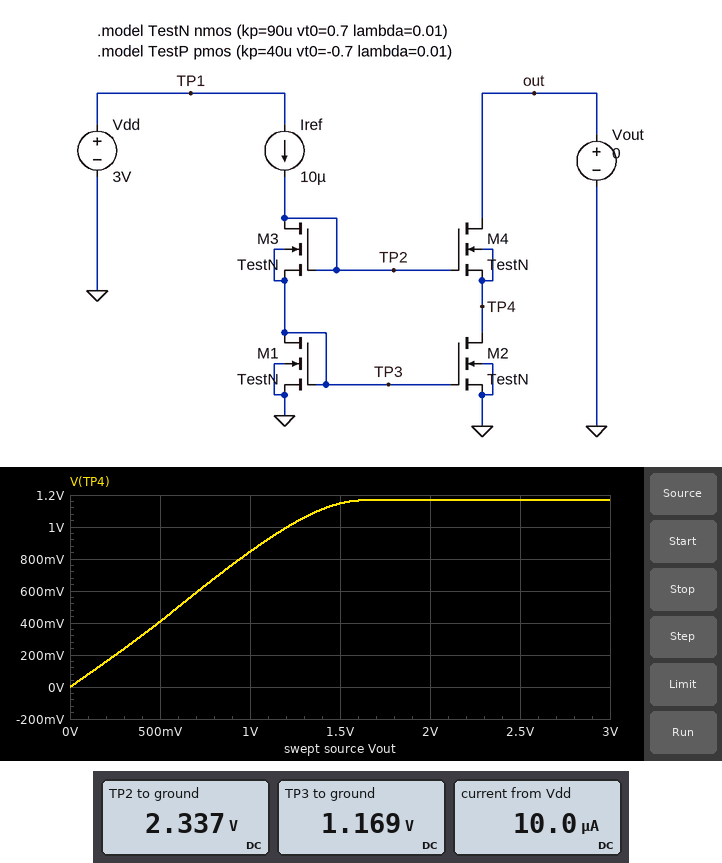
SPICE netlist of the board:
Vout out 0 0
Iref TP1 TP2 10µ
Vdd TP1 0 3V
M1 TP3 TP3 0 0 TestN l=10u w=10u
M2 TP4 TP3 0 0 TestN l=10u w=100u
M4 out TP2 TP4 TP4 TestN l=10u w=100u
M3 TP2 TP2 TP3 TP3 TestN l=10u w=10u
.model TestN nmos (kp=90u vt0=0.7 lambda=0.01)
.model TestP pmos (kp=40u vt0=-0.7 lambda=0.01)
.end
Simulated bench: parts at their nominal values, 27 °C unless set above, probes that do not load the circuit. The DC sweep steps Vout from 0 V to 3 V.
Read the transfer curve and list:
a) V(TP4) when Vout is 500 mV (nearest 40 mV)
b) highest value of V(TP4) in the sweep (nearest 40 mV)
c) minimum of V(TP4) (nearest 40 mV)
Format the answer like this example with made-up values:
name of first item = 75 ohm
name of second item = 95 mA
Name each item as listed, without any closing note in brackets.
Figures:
V(TP4) when Vout is 500 mV = 400 mV
highest value of V(TP4) in the sweep = 1.16 V
minimum of V(TP4) = 0 V
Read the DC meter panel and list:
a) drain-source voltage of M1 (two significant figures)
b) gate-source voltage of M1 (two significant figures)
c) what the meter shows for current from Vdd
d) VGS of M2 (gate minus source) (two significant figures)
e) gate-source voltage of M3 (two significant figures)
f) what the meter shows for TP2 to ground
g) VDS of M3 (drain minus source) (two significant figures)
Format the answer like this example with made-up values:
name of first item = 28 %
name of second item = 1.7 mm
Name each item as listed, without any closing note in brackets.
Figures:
drain-source voltage of M1 = 1.2 V
gate-source voltage of M1 = 1.2 V
what the meter shows for current from Vdd = 10.0 µA
VGS of M2 (gate minus source) = 1.2 V
gate-source voltage of M3 = 1.2 V
what the meter shows for TP2 to ground = 2.337 V
VDS of M3 (drain minus source) = 1.2 V
